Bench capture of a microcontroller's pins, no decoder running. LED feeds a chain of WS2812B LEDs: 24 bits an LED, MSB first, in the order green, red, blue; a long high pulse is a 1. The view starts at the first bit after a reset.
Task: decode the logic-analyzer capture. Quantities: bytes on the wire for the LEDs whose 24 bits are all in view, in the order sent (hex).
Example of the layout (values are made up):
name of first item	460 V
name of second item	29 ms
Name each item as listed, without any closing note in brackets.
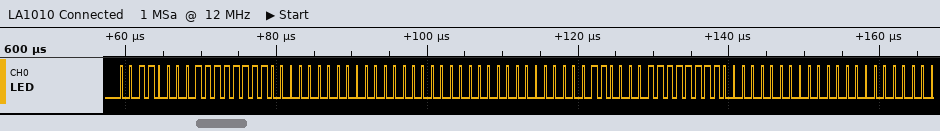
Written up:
bytes on the wire for the LEDs whose 24 bits are all in view, in the order sent	30 FF 00 00 00 00 30 FF 00
